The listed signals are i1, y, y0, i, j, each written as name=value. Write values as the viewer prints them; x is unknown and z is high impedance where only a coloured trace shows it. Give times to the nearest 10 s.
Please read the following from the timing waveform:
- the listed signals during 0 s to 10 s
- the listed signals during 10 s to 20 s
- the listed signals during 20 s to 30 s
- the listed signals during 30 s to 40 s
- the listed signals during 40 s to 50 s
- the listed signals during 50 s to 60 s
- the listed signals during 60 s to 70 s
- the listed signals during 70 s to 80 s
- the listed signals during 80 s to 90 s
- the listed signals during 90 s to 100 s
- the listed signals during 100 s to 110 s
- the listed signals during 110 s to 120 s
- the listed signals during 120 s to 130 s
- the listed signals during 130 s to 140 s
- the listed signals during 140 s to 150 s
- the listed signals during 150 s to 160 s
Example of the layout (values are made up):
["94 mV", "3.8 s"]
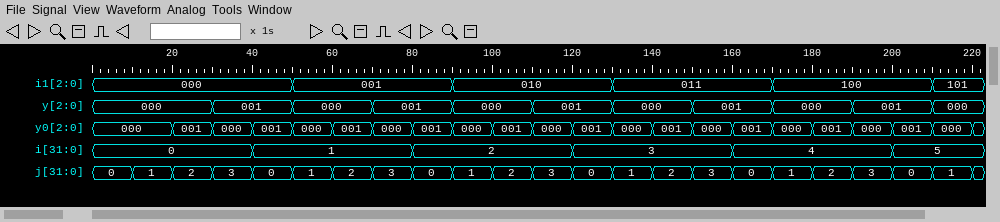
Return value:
["i1=000, y=000, y0=000, i=0, j=0", "i1=000, y=000, y0=000, i=0, j=1", "i1=000, y=000, y0=001, i=0, j=2", "i1=000, y=001, y0=000, i=0, j=3", "i1=000, y=001, y0=001, i=1, j=0", "i1=001, y=000, y0=000, i=1, j=1", "i1=001, y=000, y0=001, i=1, j=2", "i1=001, y=001, y0=000, i=1, j=3", "i1=001, y=001, y0=001, i=2, j=0", "i1=010, y=000, y0=000, i=2, j=1", "i1=010, y=000, y0=001, i=2, j=2", "i1=010, y=001, y0=000, i=2, j=3", "i1=010, y=001, y0=001, i=3, j=0", "i1=011, y=000, y0=000, i=3, j=1", "i1=011, y=000, y0=001, i=3, j=2", "i1=011, y=001, y0=000, i=3, j=3"]
